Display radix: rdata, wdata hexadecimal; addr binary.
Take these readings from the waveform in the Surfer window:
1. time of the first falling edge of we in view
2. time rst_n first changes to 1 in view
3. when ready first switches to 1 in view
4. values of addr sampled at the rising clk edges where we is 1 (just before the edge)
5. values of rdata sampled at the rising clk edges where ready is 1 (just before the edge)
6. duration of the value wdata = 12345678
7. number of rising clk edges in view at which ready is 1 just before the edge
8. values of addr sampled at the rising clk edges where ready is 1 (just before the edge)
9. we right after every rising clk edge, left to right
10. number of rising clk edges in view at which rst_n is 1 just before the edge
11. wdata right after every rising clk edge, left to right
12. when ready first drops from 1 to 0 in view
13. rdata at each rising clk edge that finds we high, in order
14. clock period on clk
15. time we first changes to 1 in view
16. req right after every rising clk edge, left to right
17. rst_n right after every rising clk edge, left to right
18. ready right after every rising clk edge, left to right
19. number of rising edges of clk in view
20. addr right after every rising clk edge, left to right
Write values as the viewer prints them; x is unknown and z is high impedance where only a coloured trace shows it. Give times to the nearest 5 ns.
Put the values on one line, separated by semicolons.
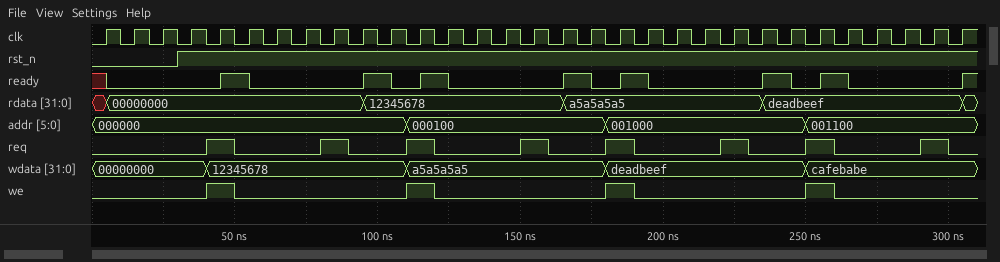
50 ns; 30 ns; 45 ns; 000000, 000100, 001000, 001100; 00000000, 12345678, 12345678, a5a5a5a5, a5a5a5a5, deadbeef, deadbeef; 70 ns; 7; 000000, 000000, 000100, 000100, 001000, 001000, 001100; 0 0 0 0 1 0 0 0 0 0 0 1 0 0 0 0 0 0 1 0 0 0 0 0 0 1 0 0 0 0 0; 28; 00000000, 00000000, 00000000, 00000000, 12345678, 12345678, 12345678, 12345678, 12345678, 12345678, 12345678, a5a5a5a5, a5a5a5a5, a5a5a5a5, a5a5a5a5, a5a5a5a5, a5a5a5a5, a5a5a5a5, deadbeef, deadbeef, deadbeef, deadbeef, deadbeef, deadbeef, deadbeef, cafebabe, cafebabe, cafebabe, cafebabe, cafebabe, cafebabe; 55 ns; 00000000, 12345678, a5a5a5a5, deadbeef; 10 ns; 40 ns; 0 0 0 0 1 0 0 0 1 0 0 1 0 0 0 1 0 0 1 0 0 0 1 0 0 1 0 0 0 1 0; 0 0 0 1 1 1 1 1 1 1 1 1 1 1 1 1 1 1 1 1 1 1 1 1 1 1 1 1 1 1 1; 0 0 0 0 1 0 0 0 0 1 0 1 0 0 0 0 1 0 1 0 0 0 0 1 0 1 0 0 0 0 1; 31; 000000, 000000, 000000, 000000, 000000, 000000, 000000, 000000, 000000, 000000, 000000, 000100, 000100, 000100, 000100, 000100, 000100, 000100, 001000, 001000, 001000, 001000, 001000, 001000, 001000, 001100, 001100, 001100, 001100, 001100, 001100
